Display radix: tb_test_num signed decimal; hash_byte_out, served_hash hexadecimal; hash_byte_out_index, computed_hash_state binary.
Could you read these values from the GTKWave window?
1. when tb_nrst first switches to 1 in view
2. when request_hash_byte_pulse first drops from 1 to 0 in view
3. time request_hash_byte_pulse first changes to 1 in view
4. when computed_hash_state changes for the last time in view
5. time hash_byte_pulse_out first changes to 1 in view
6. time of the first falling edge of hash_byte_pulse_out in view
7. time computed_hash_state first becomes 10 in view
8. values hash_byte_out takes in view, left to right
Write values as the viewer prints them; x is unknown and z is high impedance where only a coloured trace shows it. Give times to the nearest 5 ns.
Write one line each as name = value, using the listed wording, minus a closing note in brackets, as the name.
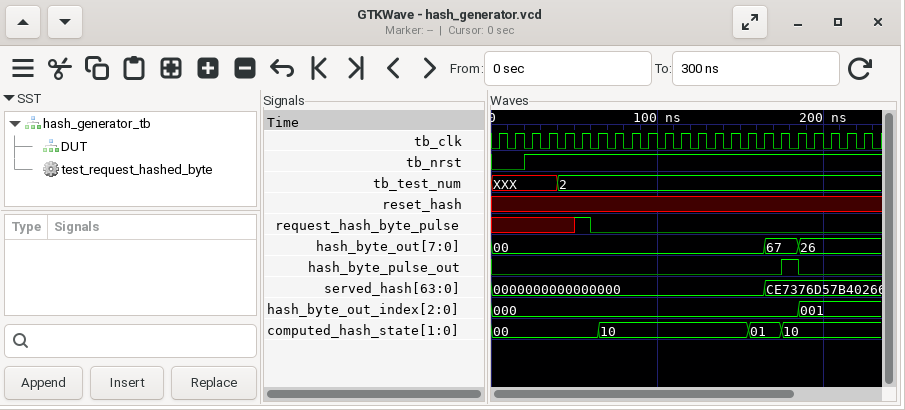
when tb_nrst first switches to 1 in view = 20 ns
when request_hash_byte_pulse first drops from 1 to 0 in view = 60 ns
time request_hash_byte_pulse first changes to 1 in view = 50 ns
when computed_hash_state changes for the last time in view = 175 ns
time hash_byte_pulse_out first changes to 1 in view = 175 ns
time of the first falling edge of hash_byte_pulse_out in view = 185 ns
time computed_hash_state first becomes 10 in view = 65 ns
values hash_byte_out takes in view, left to right = 00, 67, 26
